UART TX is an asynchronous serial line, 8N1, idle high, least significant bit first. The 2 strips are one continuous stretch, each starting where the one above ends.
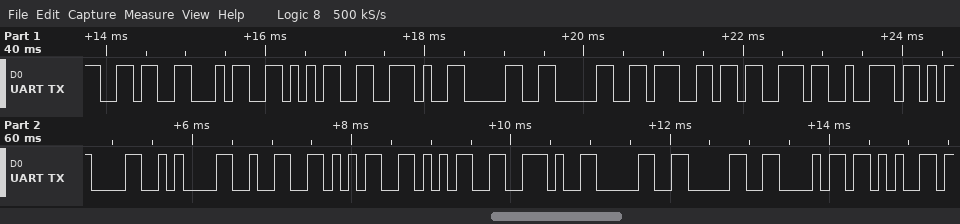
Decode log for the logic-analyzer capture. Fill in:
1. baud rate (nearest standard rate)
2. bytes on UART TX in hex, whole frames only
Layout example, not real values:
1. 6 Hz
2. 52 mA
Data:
1. 9600 baud
2. 36 34 35 2E 30 30 67 73 72 0D 0A 32 35 35 2E 30 30 68 65
